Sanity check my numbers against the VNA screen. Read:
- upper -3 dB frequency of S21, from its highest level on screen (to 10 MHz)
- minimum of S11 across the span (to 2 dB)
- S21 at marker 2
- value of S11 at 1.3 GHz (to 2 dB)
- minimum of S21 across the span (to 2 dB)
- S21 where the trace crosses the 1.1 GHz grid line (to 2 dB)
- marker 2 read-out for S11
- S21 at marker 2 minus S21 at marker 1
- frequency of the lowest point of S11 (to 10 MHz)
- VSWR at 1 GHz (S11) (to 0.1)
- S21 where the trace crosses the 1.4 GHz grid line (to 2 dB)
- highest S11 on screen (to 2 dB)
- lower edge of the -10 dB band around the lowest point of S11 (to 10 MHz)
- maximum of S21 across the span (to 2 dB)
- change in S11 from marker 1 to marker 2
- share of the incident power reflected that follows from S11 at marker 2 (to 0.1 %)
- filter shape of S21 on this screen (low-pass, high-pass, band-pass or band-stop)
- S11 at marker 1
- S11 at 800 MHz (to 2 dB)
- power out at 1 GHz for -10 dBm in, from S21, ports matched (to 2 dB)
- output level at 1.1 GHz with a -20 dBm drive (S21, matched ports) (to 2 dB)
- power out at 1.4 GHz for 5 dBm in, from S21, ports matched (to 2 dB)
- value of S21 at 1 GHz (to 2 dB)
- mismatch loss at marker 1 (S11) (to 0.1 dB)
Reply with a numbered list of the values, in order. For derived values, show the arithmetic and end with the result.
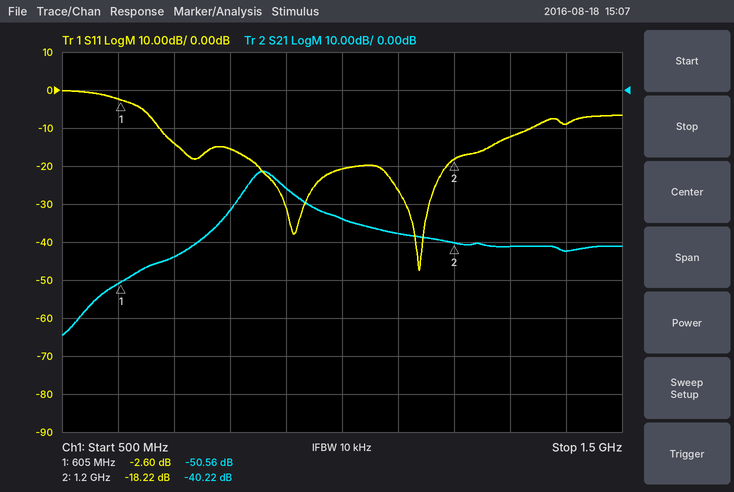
1. 890 MHz
2. -48 dB
3. -40.22 dB
4. -12 dB
5. -64 dB
6. -38 dB
7. -18.22 dB
8. -40.22 − (-50.56) = 10.34 dB
9. 1.14 GHz
10. |Γ| = 10^(-20/20) = 0.1000; VSWR = (1 + 0.1000)/(1 − 0.1000) ≈ 1.2
11. -42 dB
12. 0 dB
13. 670 MHz
14. -22 dB
15. -18.22 − (-2.6) = -15.62 dB
16. 10^(-18.22/10) ≈ 1.5 %
17. band-pass
18. -2.60 dB
19. -16 dB
20. -10 dBm + (-34 dB) = -44 dBm
21. -20 dBm + (-38 dB) = -58 dBm
22. 5 dBm + (-42 dB) = -38 dBm
23. -34 dB
24. −10 log10(1 − 10^(-2.6/10)) ≈ 3.5 dB
